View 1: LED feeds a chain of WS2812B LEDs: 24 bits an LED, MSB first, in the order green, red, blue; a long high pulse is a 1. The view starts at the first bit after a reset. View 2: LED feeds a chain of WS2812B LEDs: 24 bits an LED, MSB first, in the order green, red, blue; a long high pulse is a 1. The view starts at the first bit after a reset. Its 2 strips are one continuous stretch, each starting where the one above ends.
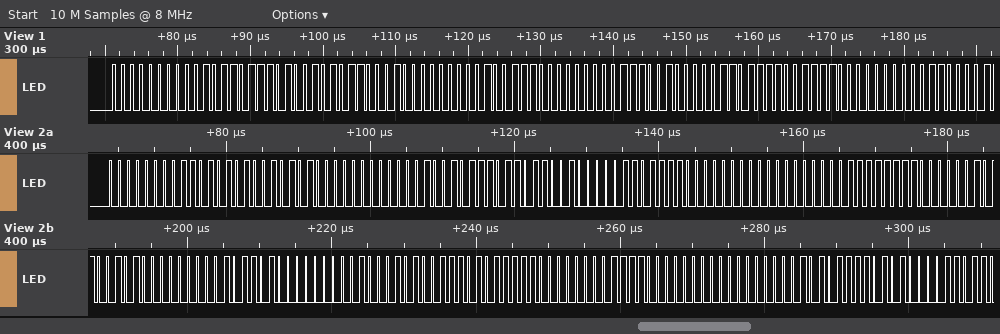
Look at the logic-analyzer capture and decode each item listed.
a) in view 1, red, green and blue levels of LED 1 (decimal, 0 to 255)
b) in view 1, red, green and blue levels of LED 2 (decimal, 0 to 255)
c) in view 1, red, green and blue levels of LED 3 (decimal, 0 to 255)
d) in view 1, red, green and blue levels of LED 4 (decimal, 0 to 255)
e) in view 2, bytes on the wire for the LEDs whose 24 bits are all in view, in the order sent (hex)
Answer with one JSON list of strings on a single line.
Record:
["45, 0, 210", "0, 177, 78", "228, 0, 27", "0, 207, 48", "00 D5 2A 00 12 ED 90 6F 00 00 3F C0 A5 00 5A 00 8A 75 F0 0F 00 00 57 A8"]
